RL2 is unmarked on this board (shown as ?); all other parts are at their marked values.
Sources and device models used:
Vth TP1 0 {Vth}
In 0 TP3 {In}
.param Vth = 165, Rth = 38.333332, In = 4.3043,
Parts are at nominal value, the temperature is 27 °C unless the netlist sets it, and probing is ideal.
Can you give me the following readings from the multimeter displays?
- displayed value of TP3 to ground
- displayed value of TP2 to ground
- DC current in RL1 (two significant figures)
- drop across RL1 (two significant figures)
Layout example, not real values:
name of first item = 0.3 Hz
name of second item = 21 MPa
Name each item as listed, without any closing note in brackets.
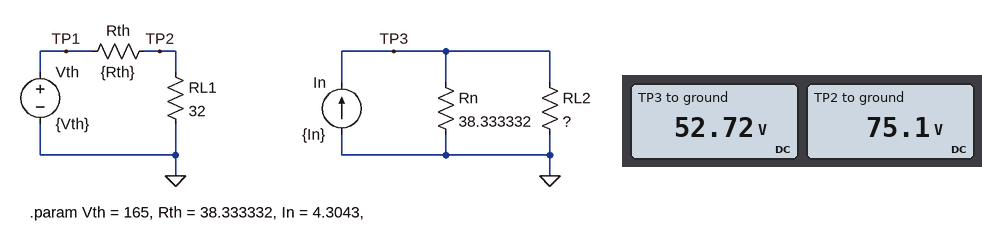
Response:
displayed value of TP3 to ground = 52.72 V
displayed value of TP2 to ground = 75.1 V
DC current in RL1 = 2.3 A
drop across RL1 = 75 V
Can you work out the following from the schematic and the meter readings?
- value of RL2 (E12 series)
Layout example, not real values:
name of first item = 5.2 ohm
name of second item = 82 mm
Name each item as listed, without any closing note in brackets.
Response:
value of RL2 = 18 Ω
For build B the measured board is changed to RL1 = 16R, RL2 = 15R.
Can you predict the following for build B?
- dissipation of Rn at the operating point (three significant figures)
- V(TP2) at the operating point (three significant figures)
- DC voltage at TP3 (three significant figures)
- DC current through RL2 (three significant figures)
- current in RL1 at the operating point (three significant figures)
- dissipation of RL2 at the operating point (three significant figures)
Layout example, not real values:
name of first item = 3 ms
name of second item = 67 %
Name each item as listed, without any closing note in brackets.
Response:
dissipation of Rn at the operating point = 56.2 W
V(TP2) at the operating point = 48.6 V
DC voltage at TP3 = 46.4 V
DC current through RL2 = 3.09 A
current in RL1 at the operating point = 3.04 A
dissipation of RL2 at the operating point = 144 W
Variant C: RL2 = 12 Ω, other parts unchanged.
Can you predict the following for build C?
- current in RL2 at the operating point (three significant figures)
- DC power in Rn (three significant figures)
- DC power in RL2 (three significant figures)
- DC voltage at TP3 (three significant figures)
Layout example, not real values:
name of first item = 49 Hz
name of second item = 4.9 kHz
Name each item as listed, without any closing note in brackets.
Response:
current in RL2 at the operating point = 3.28 A
DC power in Rn = 40.4 W
DC power in RL2 = 129 W
DC voltage at TP3 = 39.3 V
